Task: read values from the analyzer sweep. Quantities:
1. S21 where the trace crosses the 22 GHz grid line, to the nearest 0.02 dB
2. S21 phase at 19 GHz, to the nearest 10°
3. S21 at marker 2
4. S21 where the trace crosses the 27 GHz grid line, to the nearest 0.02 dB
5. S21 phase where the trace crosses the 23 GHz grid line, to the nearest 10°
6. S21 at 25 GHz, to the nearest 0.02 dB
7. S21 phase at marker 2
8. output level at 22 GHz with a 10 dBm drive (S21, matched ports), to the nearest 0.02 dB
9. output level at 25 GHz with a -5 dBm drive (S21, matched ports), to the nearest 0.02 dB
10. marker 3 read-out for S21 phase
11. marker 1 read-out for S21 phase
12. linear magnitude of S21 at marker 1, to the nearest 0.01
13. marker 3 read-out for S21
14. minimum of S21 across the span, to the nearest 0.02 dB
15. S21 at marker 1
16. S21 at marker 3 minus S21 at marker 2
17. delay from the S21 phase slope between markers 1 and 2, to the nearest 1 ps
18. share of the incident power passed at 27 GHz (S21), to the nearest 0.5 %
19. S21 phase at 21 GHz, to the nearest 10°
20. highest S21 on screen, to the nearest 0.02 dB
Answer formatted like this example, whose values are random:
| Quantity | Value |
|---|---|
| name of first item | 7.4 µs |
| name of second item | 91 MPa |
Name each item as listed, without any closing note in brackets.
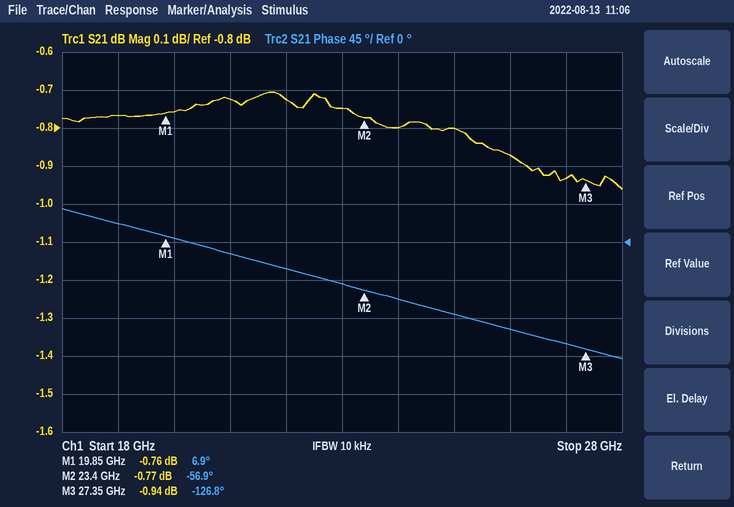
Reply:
| Quantity | Value |
|---|---|
| S21 where the trace crosses the 22 GHz grid line, to the nearest 0.02 dB | -0.72 dB |
| S21 phase at 19 GHz, to the nearest 10° | 20° |
| S21 at marker 2 | -0.77 dB |
| S21 where the trace crosses the 27 GHz grid line, to the nearest 0.02 dB | -0.94 dB |
| S21 phase where the trace crosses the 23 GHz grid line, to the nearest 10° | -50° |
| S21 at 25 GHz, to the nearest 0.02 dB | -0.80 dB |
| S21 phase at marker 2 | -56.9° |
| output level at 22 GHz with a 10 dBm drive (S21, matched ports), to the nearest 0.02 dB | 9.28 dBm |
| output level at 25 GHz with a -5 dBm drive (S21, matched ports), to the nearest 0.02 dB | -5.80 dBm |
| marker 3 read-out for S21 phase | -126.8° |
| marker 1 read-out for S21 phase | 6.9° |
| linear magnitude of S21 at marker 1, to the nearest 0.01 | 0.92 |
| marker 3 read-out for S21 | -0.94 dB |
| minimum of S21 across the span, to the nearest 0.02 dB | -0.96 dB |
| S21 at marker 1 | -0.76 dB |
| S21 at marker 3 minus S21 at marker 2 | -0.17 dB |
| delay from the S21 phase slope between markers 1 and 2, to the nearest 1 ps | 50 ps |
| share of the incident power passed at 27 GHz (S21), to the nearest 0.5 % | 80.5 % |
| S21 phase at 21 GHz, to the nearest 10° | -10° |
| highest S21 on screen, to the nearest 0.02 dB | -0.70 dB |
